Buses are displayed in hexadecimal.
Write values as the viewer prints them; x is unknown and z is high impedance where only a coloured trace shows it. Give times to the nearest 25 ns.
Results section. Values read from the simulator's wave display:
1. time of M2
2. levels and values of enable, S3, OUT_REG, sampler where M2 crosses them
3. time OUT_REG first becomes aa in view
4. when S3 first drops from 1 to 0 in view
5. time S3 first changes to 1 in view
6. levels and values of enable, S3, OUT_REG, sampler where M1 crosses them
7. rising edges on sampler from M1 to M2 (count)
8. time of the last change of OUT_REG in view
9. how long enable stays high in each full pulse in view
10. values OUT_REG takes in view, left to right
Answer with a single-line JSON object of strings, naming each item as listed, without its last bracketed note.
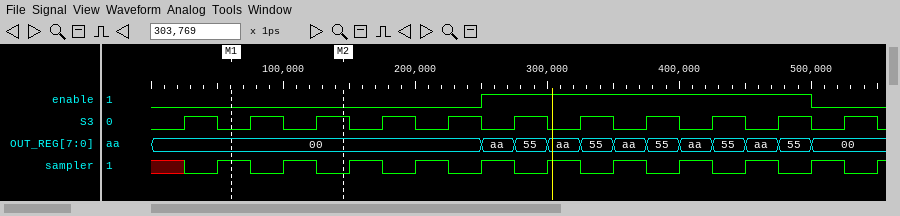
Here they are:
{"time of M2": "150 ns", "levels and values of enable, S3, OUT_REG, sampler where M2 crosses them": "enable=0, S3=1, OUT_REG=00, sampler=0", "time OUT_REG first becomes aa in view": "250 ns", "when S3 first drops from 1 to 0 in view": "50 ns", "time S3 first changes to 1 in view": "25 ns", "levels and values of enable, S3, OUT_REG, sampler where M1 crosses them": "enable=0, S3=0, OUT_REG=00, sampler=1", "rising edges on sampler from M1 to M2": "1", "time of the last change of OUT_REG in view": "500 ns", "how long enable stays high in each full pulse in view": "250 ns", "values OUT_REG takes in view, left to right": "00, aa, 55, aa, 55, aa, 55, aa, 55, aa, 55, 00"}
